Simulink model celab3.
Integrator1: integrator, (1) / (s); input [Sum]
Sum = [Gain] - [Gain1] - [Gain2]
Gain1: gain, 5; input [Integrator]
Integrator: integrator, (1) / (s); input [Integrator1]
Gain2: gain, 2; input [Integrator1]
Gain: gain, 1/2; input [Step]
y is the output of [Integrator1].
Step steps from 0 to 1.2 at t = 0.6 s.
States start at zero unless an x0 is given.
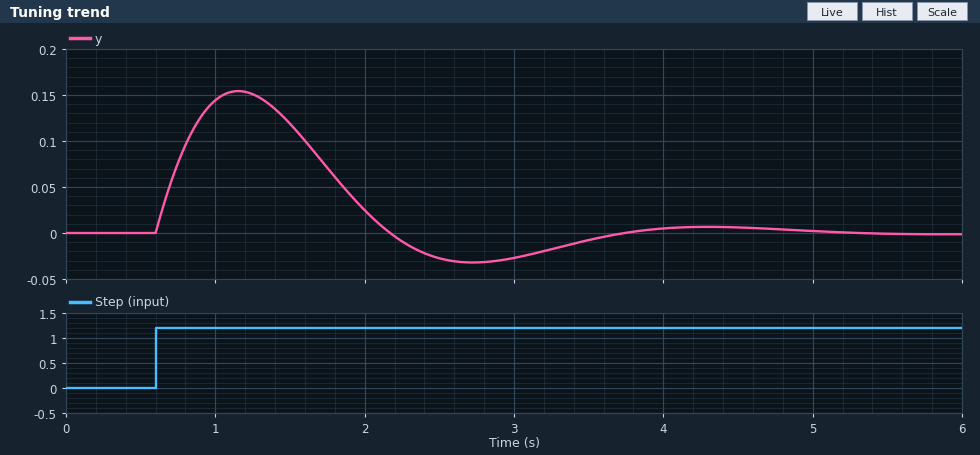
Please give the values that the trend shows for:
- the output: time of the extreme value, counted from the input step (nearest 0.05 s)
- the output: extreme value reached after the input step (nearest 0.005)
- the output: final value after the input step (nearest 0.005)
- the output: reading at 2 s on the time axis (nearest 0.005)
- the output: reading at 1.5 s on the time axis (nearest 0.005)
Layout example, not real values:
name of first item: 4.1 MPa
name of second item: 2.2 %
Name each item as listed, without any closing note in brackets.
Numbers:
the output: time of the extreme value, counted from the input step: 0.55 s
the output: extreme value reached after the input step: 0.155
the output: final value after the input step: 0.000
the output: reading at 2 s on the time axis: 0.025
the output: reading at 1.5 s on the time axis: 0.120
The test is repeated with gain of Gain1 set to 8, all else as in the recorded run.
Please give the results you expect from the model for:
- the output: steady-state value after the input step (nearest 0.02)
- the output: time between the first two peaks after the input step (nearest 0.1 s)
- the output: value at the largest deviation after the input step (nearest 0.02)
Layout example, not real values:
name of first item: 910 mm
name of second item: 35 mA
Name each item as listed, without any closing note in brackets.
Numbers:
the output: steady-state value after the input step: 0.00
the output: time between the first two peaks after the input step: 2.4 s
the output: value at the largest deviation after the input step: 0.14
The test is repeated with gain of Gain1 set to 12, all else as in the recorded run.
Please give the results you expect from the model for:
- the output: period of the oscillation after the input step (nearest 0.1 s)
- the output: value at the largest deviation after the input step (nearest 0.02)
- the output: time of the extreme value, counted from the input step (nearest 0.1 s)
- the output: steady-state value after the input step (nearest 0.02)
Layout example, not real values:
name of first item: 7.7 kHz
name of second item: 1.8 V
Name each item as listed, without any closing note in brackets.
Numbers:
the output: period of the oscillation after the input step: 1.9 s
the output: value at the largest deviation after the input step: 0.12
the output: time of the extreme value, counted from the input step: 0.4 s
the output: steady-state value after the input step: 0.00
